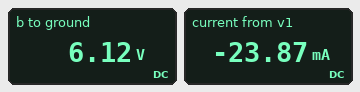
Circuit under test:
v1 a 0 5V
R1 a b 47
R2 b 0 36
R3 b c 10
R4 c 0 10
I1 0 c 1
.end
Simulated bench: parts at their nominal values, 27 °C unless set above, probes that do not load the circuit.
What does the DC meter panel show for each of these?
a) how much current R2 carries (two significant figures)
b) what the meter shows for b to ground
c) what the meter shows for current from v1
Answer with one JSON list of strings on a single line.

["170 mA", "6.12 V", "-23.87 mA"]
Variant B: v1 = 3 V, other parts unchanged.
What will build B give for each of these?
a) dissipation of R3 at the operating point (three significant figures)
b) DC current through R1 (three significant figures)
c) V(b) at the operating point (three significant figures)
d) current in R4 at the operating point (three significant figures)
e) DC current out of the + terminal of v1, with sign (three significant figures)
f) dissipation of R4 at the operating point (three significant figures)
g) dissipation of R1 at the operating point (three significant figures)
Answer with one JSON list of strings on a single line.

["464 mW", "57.3 mA", "5.69 V", "785 mA", "-57.3 mA", "6.16 W", "154 mW"]
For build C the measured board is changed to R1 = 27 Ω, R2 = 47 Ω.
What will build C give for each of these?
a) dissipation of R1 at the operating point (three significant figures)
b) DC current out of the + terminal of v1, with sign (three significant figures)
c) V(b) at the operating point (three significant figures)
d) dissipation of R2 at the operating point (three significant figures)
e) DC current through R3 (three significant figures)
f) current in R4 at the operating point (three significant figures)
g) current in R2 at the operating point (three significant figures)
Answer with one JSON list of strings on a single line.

["65.1 mW", "-49.1 mA", "6.33 V", "851 mW", "184 mA", "816 mA", "135 mA"]
